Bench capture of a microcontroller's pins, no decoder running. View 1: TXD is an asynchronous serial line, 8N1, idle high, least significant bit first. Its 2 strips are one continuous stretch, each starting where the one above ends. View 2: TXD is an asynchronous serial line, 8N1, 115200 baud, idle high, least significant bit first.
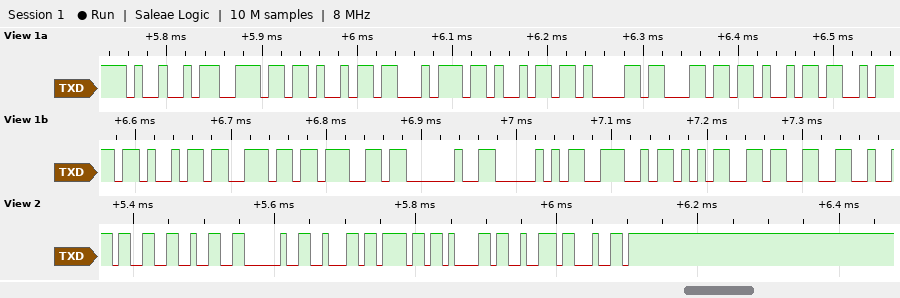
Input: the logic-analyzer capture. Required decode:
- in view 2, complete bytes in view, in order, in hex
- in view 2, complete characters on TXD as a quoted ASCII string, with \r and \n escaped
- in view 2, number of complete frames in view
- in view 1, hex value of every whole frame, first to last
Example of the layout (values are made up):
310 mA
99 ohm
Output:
33 32 20 62 6F 61 72 64
"32 board"
8
0x49 0x6E 0x69 0x74 0x69 0x61 0x6C 0x69 0x7A 0x69 0x6E 0x67 0x20 0x50 0x4E 0x35 0x33
